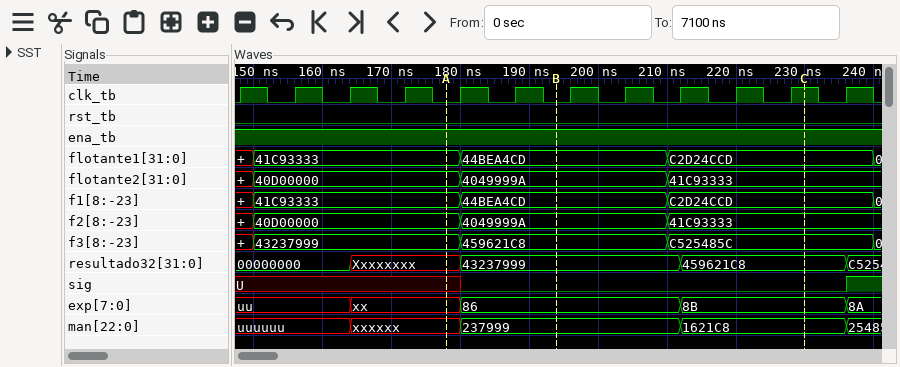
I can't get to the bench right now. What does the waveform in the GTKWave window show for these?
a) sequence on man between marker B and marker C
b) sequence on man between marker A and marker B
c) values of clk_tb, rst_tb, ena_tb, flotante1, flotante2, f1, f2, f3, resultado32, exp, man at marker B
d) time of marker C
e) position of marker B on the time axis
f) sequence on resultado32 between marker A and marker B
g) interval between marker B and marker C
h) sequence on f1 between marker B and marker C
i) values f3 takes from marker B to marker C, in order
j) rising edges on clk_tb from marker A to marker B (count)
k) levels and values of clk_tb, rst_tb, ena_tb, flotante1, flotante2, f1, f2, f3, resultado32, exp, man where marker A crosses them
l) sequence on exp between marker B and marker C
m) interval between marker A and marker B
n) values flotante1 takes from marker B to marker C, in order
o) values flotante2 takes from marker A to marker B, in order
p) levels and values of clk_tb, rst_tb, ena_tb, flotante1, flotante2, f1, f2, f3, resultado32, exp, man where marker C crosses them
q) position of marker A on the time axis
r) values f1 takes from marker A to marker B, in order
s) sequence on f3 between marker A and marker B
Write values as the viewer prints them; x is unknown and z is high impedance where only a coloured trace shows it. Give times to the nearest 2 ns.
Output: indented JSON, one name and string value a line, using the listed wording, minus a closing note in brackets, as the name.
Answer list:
{
  "sequence on man between marker B and marker C": "237999, 1621C8",
  "sequence on man between marker A and marker B": "xxxxxx, 237999",
  "values of clk_tb, rst_tb, ena_tb, flotante1, flotante2, f1, f2, f3, resultado32, exp, man at marker B": "clk_tb=0, rst_tb=0, ena_tb=1, flotante1=44BEA4CD, flotante2=4049999A, f1=44BEA4CD, f2=4049999A, f3=459621C8, resultado32=43237999, exp=86, man=237999",
  "time of marker C": "230 ns",
  "position of marker B on the time axis": "194 ns",
  "sequence on resultado32 between marker A and marker B": "Xxxxxxxx, 43237999",
  "interval between marker B and marker C": "36 ns",
  "sequence on f1 between marker B and marker C": "44BEA4CD, C2D24CCD",
  "values f3 takes from marker B to marker C, in order": "459621C8, C525485C",
  "rising edges on clk_tb from marker A to marker B": "2",
  "levels and values of clk_tb, rst_tb, ena_tb, flotante1, flotante2, f1, f2, f3, resultado32, exp, man where marker A crosses them": "clk_tb=0, rst_tb=0, ena_tb=1, flotante1=41C93333, flotante2=40D00000, f1=41C93333, f2=40D00000, f3=43237999, resultado32=Xxxxxxxx, exp=xx, man=xxxxxx",
  "sequence on exp between marker B and marker C": "86, 8B",
  "interval between marker A and marker B": "16 ns",
  "values flotante1 takes from marker B to marker C, in order": "44BEA4CD, C2D24CCD",
  "values flotante2 takes from marker A to marker B, in order": "40D00000, 4049999A",
  "levels and values of clk_tb, rst_tb, ena_tb, flotante1, flotante2, f1, f2, f3, resultado32, exp, man where marker C crosses them": "clk_tb=1, rst_tb=0, ena_tb=1, flotante1=C2D24CCD, flotante2=41C93333, f1=C2D24CCD, f2=41C93333, f3=C525485C, resultado32=459621C8, exp=8B, man=1621C8",
  "position of marker A on the time axis": "178 ns",
  "values f1 takes from marker A to marker B, in order": "41C93333, 44BEA4CD",
  "sequence on f3 between marker A and marker B": "43237999, 459621C8"
}
